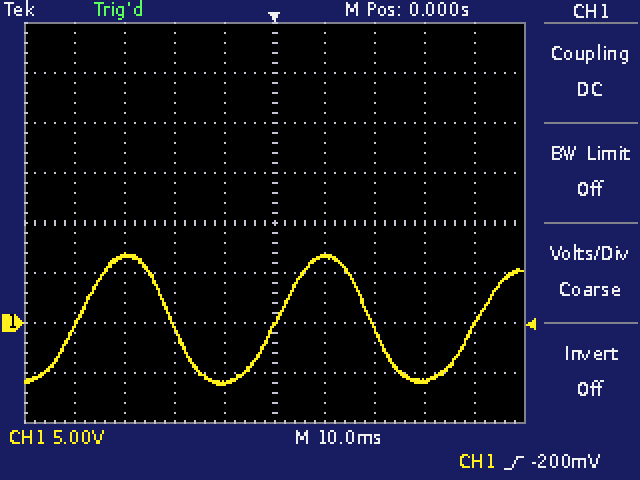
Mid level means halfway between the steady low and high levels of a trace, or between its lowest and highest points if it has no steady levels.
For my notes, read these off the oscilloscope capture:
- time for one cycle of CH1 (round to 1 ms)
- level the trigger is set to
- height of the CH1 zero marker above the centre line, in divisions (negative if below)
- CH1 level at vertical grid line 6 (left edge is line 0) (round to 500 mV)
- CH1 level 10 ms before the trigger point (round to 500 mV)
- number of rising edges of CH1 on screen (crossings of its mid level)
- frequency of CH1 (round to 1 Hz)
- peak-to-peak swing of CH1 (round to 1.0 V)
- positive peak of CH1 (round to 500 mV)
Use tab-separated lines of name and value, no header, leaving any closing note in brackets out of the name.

time for one cycle of CH1	40 ms
level the trigger is set to	-200 mV
height of the CH1 zero marker above the centre line, in divisions	-2.0 div
CH1 level at vertical grid line 6 (left edge is line 0)	6.5 V
CH1 level 10 ms before the trigger point	-6.0 V
number of rising edges of CH1 on screen	3
frequency of CH1	25 Hz
peak-to-peak swing of CH1	13.0 V
positive peak of CH1	7.0 V
